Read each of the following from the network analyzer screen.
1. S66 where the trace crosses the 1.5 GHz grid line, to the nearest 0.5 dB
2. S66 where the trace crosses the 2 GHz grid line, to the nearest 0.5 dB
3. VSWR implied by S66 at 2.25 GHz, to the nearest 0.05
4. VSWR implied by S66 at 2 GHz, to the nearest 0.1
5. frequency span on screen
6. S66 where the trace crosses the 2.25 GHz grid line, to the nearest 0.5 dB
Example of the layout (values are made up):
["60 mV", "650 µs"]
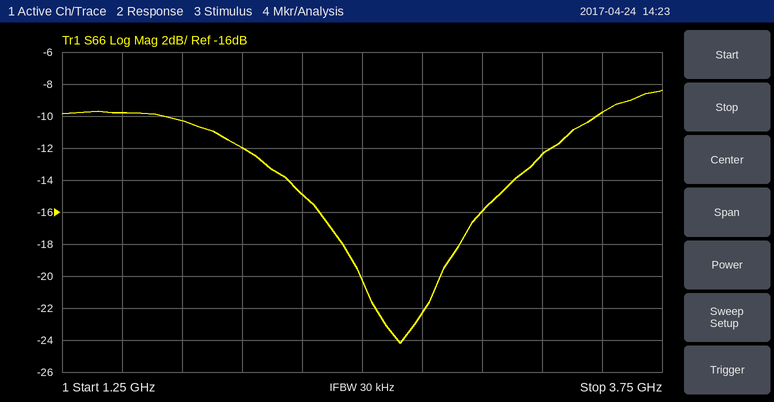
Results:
["-10.0 dB", "-12.0 dB", "1.45", "1.7", "2.5 GHz", "-15.0 dB"]
